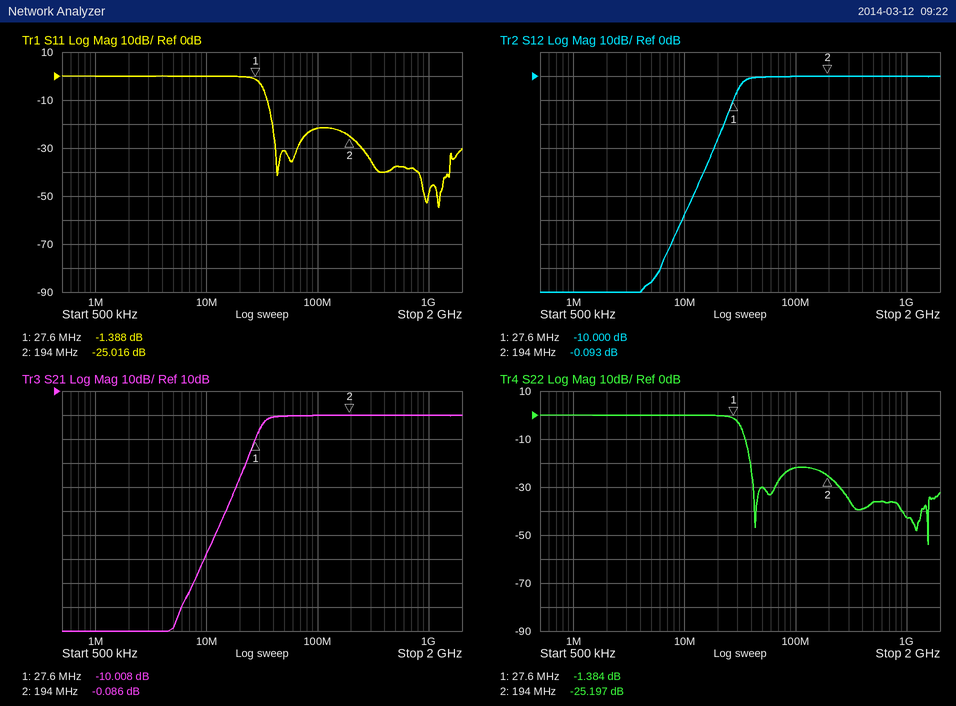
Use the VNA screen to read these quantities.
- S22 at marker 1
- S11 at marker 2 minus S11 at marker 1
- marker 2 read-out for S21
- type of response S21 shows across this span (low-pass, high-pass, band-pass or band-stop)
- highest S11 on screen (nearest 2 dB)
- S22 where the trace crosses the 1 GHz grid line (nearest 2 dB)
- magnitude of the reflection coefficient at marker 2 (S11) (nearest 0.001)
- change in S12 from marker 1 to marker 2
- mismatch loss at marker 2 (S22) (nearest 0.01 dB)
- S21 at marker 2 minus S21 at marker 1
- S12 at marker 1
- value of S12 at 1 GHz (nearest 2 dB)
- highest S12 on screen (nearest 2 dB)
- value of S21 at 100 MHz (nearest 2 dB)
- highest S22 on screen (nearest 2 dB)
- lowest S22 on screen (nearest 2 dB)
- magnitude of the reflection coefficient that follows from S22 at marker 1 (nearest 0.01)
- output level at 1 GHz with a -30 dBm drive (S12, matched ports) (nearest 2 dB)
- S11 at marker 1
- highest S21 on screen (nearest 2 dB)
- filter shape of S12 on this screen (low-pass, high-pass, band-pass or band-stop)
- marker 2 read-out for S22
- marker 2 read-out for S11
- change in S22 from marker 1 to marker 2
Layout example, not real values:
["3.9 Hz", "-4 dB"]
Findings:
["-1.384 dB", "-23.628 dB", "-0.086 dB", "high-pass", "0 dB", "-42 dB", "0.056", "9.907 dB", "0.01 dB", "9.922 dB", "-10.000 dB", "0 dB", "0 dB", "0 dB", "0 dB", "-54 dB", "0.85", "-30 dBm", "-1.388 dB", "0 dB", "high-pass", "-25.197 dB", "-25.016 dB", "-23.813 dB"]
